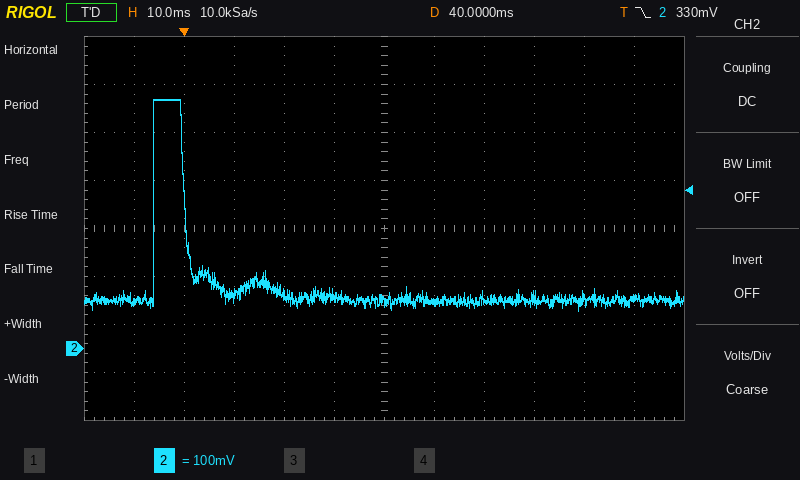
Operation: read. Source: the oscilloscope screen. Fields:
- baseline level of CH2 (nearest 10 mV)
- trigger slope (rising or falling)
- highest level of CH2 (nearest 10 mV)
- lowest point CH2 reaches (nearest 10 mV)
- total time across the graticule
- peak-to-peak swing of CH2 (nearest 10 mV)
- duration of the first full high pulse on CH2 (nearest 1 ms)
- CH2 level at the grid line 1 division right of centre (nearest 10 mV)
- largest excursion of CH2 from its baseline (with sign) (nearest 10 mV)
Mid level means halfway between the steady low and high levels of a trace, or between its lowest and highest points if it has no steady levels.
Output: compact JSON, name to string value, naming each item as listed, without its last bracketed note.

{"baseline level of CH2": "100 mV", "trigger slope": "falling", "highest level of CH2": "520 mV", "lowest point CH2 reaches": "80 mV", "total time across the graticule": "120 ms", "peak-to-peak swing of CH2": "440 mV", "duration of the first full high pulse on CH2": "6 ms", "CH2 level at the grid line 1 division right of centre": "100 mV", "largest excursion of CH2 from its baseline (with sign)": "+420 mV"}
